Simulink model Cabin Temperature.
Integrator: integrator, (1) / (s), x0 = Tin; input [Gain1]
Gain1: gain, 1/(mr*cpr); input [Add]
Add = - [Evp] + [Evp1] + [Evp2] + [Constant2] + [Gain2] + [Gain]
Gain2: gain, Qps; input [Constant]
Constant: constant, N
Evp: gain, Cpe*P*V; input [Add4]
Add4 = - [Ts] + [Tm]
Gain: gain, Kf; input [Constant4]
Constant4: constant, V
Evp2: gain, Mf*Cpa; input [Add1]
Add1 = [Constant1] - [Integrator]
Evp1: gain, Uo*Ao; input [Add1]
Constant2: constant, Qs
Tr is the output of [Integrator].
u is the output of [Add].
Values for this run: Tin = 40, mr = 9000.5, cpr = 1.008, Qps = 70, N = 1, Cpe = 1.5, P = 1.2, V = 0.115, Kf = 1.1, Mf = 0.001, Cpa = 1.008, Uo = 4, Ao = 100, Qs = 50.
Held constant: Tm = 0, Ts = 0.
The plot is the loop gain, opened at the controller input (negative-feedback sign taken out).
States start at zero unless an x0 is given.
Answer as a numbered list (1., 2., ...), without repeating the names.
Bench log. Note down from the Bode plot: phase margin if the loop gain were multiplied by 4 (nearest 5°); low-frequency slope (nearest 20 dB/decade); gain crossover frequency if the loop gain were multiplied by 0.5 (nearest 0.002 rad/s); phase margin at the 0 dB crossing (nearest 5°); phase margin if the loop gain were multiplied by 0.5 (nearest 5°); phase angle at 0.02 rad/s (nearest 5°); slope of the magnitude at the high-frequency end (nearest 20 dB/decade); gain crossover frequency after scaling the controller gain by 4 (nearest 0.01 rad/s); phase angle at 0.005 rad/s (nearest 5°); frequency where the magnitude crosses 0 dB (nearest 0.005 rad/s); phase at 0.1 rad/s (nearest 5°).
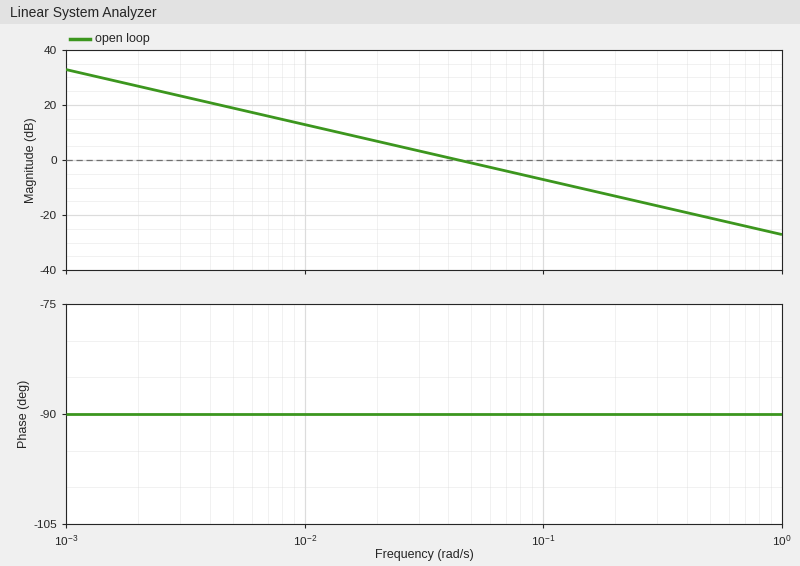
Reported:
1. 90°
2. -20 dB/decade
3. 0.022 rad/s
4. 90°
5. 90°
6. -90°
7. -20 dB/decade
8. 0.18 rad/s
9. -90°
10. 0.045 rad/s
11. -90°
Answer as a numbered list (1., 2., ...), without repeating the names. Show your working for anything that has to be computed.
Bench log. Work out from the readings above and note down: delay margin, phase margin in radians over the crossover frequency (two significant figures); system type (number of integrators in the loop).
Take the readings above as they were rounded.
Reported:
1. 90 × π / 180 / 0.045 = 35 s
2. 1
